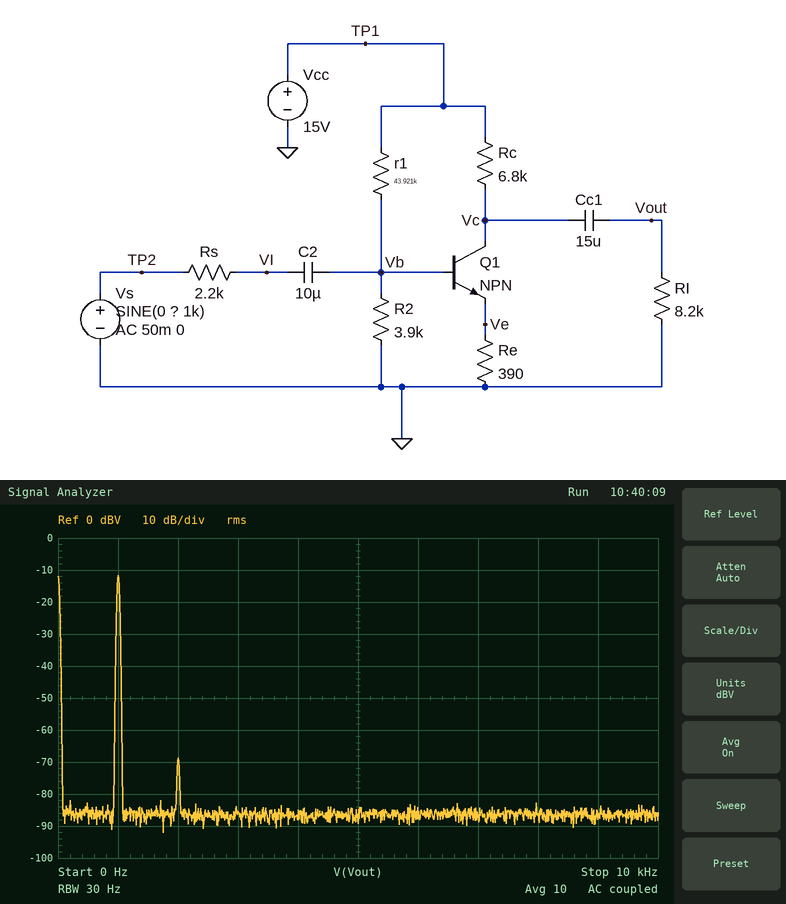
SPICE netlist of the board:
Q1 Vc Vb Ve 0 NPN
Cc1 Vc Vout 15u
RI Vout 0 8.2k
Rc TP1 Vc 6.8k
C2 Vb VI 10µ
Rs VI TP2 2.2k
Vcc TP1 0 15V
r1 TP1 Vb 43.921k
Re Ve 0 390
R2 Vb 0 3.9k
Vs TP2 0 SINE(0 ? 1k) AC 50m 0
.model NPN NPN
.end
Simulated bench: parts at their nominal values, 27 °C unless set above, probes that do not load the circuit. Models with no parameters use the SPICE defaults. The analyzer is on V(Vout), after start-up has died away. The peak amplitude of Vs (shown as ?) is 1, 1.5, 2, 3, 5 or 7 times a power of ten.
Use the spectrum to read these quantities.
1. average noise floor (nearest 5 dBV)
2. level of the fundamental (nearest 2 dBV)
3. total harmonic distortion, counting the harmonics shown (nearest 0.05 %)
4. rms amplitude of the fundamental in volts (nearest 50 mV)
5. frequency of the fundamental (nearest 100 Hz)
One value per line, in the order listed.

-85 dBV
-12 dBV
0.15 %
250 mV
1.0 kHz
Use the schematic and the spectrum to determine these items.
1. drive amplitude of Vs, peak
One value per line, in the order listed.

70 mV
